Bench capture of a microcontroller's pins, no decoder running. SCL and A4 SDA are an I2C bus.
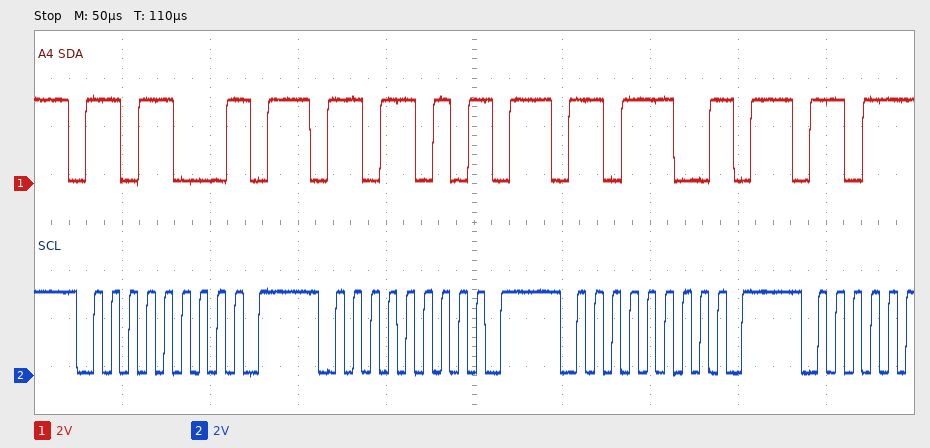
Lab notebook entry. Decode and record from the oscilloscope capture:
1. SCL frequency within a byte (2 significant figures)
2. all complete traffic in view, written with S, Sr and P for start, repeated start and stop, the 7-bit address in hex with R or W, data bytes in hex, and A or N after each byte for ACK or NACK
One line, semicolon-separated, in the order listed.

100 kHz; S 6CW N P S 6DW N P S 6EW N P
